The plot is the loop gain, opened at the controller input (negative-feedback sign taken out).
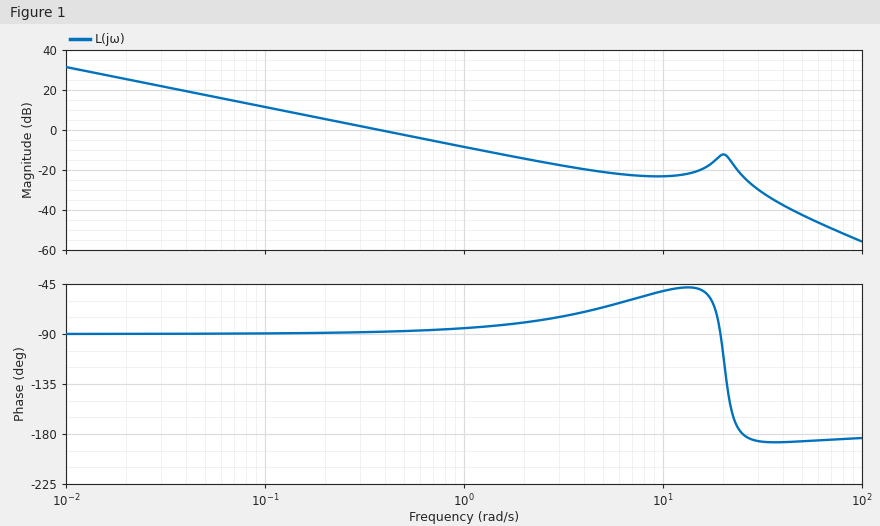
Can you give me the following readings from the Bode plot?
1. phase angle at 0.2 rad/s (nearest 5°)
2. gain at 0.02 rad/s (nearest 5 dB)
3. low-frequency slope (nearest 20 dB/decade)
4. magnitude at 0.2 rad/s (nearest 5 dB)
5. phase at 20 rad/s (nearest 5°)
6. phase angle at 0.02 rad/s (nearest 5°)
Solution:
-90°
25 dB
-20 dB/decade
5 dB
-105°
-90°
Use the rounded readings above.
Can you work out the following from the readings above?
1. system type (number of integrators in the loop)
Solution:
1
